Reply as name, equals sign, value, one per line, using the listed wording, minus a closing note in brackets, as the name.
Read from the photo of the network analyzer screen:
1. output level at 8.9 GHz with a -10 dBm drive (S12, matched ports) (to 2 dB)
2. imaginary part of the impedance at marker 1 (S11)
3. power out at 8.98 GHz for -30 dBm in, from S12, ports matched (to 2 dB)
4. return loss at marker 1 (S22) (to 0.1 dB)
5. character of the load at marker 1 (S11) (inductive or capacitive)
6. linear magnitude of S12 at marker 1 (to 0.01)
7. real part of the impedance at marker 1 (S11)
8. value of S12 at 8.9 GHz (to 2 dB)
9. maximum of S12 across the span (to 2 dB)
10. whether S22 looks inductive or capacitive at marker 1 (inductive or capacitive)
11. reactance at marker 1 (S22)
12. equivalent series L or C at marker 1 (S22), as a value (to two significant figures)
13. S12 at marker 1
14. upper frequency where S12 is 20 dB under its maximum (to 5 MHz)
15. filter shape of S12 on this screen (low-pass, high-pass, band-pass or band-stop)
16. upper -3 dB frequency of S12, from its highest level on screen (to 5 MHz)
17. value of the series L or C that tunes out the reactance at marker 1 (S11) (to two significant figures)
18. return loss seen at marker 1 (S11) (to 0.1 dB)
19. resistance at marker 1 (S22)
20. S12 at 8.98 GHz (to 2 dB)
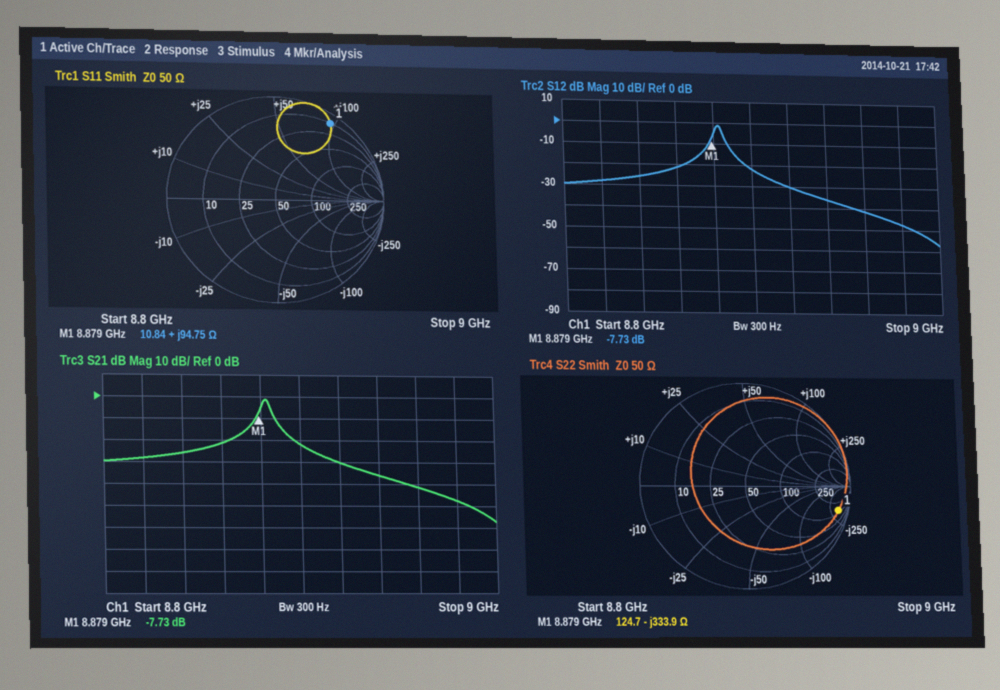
output level at 8.9 GHz with a -10 dBm drive (S12, matched ports) = -32 dBm
imaginary part of the impedance at marker 1 = +94.75 Ω
power out at 8.98 GHz for -30 dBm in, from S12, ports matched = -78 dBm
return loss at marker 1 (S22) = 0.8 dB
character of the load at marker 1 (S11) = inductive
linear magnitude of S12 at marker 1 = 0.41
real part of the impedance at marker 1 = 10.84 Ω
value of S12 at 8.9 GHz = -22 dB
maximum of S12 across the span = -2 dB
whether S22 looks inductive or capacitive at marker 1 = capacitive
reactance at marker 1 = -333.9 Ω
equivalent series L or C at marker 1 (S22), as a value = 54 fF
S12 at marker 1 = -7.73 dB
upper frequency where S12 is 20 dB under its maximum = 8.900 GHz
filter shape of S12 on this screen = band-pass
upper -3 dB frequency of S12, from its highest level on screen = 8.885 GHz
value of the series L or C that tunes out the reactance at marker 1 (S11) = 190 fF
return loss seen at marker 1 (S11) = 0.8 dB
resistance at marker 1 = 124.7 Ω
S12 at 8.98 GHz = -48 dB
